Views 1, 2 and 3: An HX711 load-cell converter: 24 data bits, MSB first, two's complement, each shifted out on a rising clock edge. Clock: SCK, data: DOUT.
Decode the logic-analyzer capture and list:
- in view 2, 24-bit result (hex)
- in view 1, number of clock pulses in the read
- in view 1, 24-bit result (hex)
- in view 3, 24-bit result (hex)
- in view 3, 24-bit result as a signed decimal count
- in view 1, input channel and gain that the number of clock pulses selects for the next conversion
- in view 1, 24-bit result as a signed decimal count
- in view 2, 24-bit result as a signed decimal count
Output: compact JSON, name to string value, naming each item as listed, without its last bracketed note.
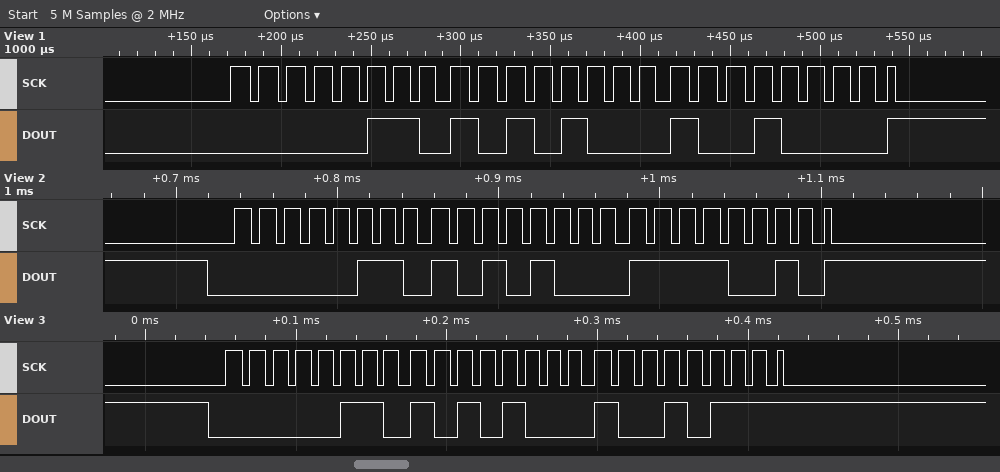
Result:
{"in view 2, 24-bit result": "0x06A8F2", "in view 1, number of clock pulses in the read": "25", "in view 1, 24-bit result": "0x06A890", "in view 3, 24-bit result": "0x06A897", "in view 3, 24-bit result as a signed decimal count": "436375", "in view 1, input channel and gain that the number of clock pulses selects for the next conversion": "channel A, gain 128", "in view 1, 24-bit result as a signed decimal count": "436368", "in view 2, 24-bit result as a signed decimal count": "436466"}
